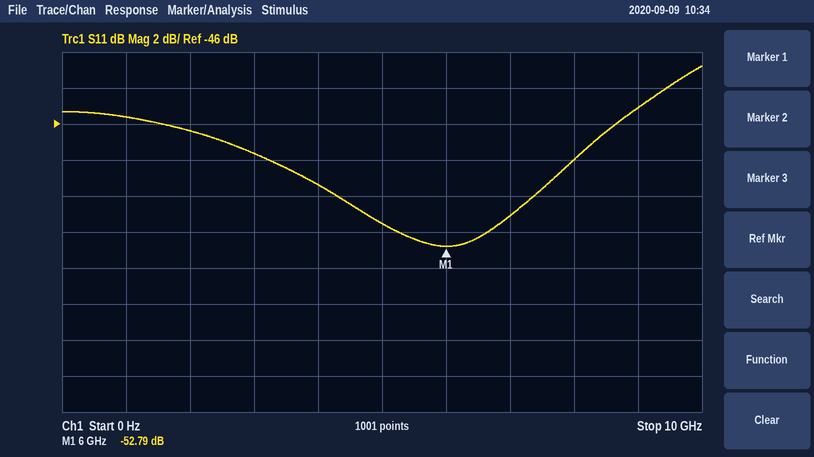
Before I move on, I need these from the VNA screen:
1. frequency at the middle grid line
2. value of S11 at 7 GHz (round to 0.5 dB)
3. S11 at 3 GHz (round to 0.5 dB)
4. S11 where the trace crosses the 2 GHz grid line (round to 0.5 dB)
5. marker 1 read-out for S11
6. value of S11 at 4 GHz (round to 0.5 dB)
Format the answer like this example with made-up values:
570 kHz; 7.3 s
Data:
5 GHz; -51.0 dB; -47.5 dB; -46.5 dB; -52.79 dB; -49.5 dB
